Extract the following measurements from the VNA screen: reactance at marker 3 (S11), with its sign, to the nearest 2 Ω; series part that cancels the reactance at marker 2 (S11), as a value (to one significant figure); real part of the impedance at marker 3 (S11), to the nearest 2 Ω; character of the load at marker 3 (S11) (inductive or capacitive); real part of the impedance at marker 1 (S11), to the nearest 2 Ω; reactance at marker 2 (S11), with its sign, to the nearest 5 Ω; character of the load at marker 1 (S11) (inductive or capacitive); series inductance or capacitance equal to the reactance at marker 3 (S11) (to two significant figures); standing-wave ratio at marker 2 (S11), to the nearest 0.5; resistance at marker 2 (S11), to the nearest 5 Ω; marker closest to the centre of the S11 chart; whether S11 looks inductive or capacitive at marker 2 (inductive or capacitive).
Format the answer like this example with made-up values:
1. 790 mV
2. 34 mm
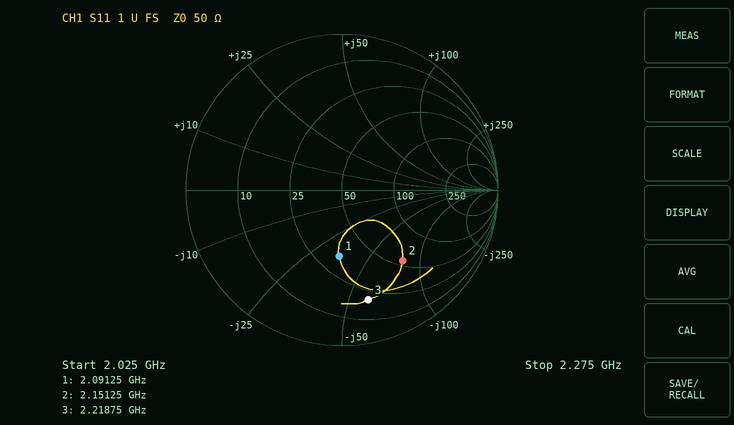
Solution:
1. -60 Ω
2. 6 nH
3. 20 Ω
4. capacitive
5. 34 Ω
6. -80 Ω
7. capacitive
8. 1.2 pF
9. 4.0
10. 55 Ω
11. marker 1
12. capacitive
